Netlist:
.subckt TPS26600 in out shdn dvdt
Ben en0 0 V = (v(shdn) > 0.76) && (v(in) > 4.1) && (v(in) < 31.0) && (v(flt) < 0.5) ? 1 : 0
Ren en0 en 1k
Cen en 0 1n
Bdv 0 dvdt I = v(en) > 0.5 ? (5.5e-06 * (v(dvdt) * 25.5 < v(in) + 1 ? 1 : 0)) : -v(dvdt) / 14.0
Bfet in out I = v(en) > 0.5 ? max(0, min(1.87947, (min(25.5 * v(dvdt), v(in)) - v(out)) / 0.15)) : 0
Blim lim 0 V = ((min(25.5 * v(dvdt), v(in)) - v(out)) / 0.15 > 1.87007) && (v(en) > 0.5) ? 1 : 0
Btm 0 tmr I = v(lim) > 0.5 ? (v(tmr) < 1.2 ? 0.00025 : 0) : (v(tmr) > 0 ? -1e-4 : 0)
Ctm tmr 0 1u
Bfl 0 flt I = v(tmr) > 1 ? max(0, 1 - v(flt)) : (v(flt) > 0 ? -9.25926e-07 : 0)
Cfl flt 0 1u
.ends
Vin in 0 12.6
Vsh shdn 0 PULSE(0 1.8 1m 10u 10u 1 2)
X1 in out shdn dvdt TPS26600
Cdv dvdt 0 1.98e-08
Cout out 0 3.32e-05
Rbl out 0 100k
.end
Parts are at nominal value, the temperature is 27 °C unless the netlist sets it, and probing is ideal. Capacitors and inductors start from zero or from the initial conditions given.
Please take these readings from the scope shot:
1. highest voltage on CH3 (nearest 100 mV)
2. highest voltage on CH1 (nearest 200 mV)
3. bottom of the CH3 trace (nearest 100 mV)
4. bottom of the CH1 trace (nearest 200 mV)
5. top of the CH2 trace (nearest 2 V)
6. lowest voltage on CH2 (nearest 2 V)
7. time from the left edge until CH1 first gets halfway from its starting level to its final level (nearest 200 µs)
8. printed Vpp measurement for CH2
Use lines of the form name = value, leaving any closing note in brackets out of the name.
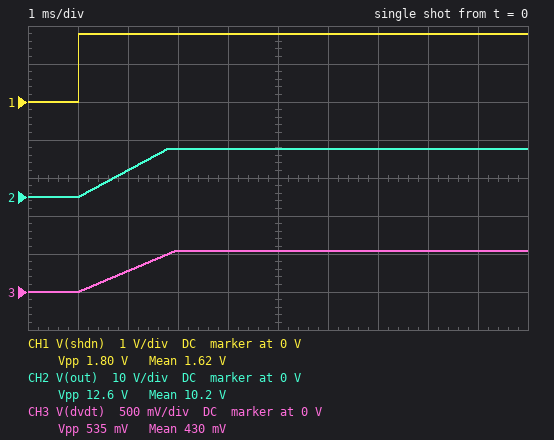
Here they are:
highest voltage on CH3 = 500 mV
highest voltage on CH1 = 1.8 V
bottom of the CH3 trace = 0 V
bottom of the CH1 trace = 0 V
top of the CH2 trace = 12 V
lowest voltage on CH2 = 0 V
time from the left edge until CH1 first gets halfway from its starting level to its final level = 1.0 ms
printed Vpp measurement for CH2 = 12.6 V
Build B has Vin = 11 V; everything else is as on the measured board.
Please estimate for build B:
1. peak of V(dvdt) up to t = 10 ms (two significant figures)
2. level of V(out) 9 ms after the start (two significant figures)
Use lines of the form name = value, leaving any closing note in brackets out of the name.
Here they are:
peak of V(dvdt) up to t = 10 ms = 470 mV
level of V(out) 9 ms after the start = 11 V
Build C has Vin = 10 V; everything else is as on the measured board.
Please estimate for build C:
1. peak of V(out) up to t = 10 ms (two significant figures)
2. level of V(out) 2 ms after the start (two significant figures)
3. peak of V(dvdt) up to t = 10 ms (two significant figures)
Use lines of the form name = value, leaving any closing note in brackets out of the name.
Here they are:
peak of V(out) up to t = 10 ms = 10 V
level of V(out) 2 ms after the start = 7.0 V
peak of V(dvdt) up to t = 10 ms = 430 mV
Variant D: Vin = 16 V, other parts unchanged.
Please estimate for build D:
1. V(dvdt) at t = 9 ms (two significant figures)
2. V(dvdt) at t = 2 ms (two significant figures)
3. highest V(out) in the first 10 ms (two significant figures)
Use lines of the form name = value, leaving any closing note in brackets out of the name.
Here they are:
V(dvdt) at t = 9 ms = 670 mV
V(dvdt) at t = 2 ms = 280 mV
highest V(out) in the first 10 ms = 16 V
